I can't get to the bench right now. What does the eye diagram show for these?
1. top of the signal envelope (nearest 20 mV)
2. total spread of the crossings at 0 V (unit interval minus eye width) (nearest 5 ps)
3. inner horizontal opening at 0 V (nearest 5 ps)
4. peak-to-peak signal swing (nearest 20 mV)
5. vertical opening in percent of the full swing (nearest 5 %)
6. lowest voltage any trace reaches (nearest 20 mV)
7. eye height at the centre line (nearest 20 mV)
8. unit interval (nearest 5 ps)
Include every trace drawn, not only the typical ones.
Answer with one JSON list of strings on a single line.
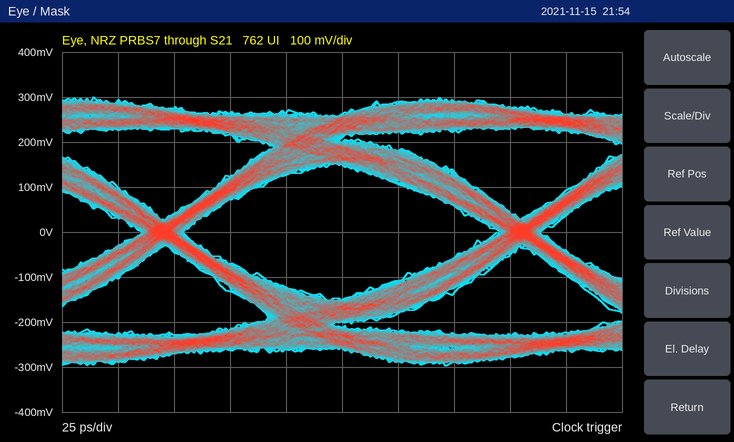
["300 mV", "20 ps", "140 ps", "600 mV", "50 %", "-300 mV", "300 mV", "160 ps"]
